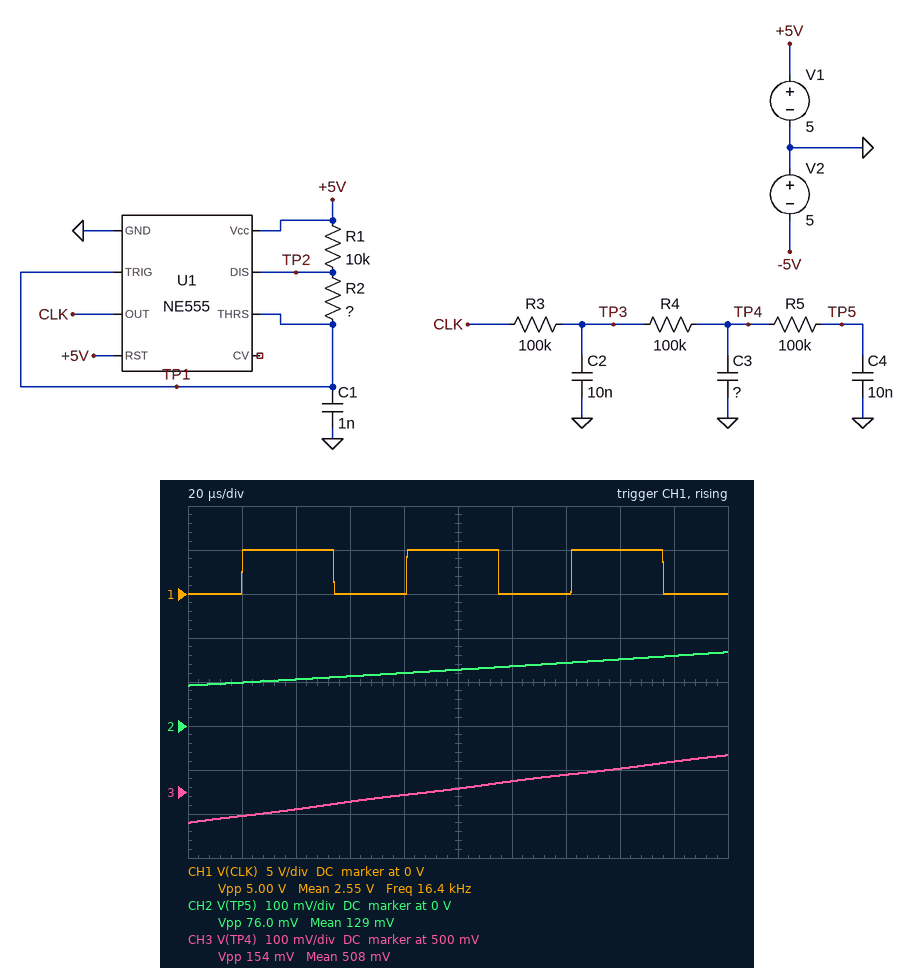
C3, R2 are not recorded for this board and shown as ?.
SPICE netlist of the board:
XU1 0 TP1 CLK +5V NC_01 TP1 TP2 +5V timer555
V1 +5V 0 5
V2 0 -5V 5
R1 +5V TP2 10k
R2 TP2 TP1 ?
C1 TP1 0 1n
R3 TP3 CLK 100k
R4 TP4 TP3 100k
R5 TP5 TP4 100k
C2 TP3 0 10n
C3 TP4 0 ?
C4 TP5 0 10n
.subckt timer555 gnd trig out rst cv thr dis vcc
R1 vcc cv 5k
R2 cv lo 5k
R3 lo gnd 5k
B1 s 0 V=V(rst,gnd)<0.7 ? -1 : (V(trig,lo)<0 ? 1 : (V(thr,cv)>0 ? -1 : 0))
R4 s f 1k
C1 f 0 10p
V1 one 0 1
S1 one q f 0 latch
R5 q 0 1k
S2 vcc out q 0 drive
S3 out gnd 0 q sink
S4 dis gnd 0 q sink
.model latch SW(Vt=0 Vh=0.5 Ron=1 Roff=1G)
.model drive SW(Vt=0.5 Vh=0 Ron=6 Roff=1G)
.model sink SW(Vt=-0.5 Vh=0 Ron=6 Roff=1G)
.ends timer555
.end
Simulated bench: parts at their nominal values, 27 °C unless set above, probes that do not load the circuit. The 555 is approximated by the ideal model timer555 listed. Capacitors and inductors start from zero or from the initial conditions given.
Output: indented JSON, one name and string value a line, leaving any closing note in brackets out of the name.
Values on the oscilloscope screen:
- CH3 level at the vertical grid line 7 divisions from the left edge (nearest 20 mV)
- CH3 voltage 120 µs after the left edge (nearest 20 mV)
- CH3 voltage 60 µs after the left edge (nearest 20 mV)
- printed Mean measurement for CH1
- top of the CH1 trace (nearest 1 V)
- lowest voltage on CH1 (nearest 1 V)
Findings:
{
  "CH3 level at the vertical grid line 7 divisions from the left edge": "540 mV",
  "CH3 voltage 120 µs after the left edge": "520 mV",
  "CH3 voltage 60 µs after the left edge": "480 mV",
  "printed Mean measurement for CH1": "2.55 V",
  "top of the CH1 trace": "5 V",
  "lowest voltage on CH1": "0 V"
}
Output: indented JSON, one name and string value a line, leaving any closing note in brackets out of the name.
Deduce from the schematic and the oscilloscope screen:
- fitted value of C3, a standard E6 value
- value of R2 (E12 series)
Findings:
{
  "fitted value of C3, a standard E6 value": "3.3 nF",
  "value of R2": "39 kΩ"
}
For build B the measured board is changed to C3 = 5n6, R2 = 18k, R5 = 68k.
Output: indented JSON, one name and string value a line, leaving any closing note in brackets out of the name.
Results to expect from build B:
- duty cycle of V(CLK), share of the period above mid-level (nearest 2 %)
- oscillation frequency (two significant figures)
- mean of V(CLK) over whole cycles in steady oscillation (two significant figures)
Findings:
{
  "duty cycle of V(CLK), share of the period above mid-level": "60 %",
  "oscillation frequency": "31 kHz",
  "mean of V(CLK) over whole cycles in steady oscillation": "3.0 V"
}
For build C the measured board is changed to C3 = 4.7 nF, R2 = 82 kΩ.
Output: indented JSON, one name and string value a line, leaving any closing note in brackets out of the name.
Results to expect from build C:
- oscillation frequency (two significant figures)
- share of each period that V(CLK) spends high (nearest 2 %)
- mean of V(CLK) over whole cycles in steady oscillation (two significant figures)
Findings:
{
  "oscillation frequency": "8.3 kHz",
  "share of each period that V(CLK) spends high": "52 %",
  "mean of V(CLK) over whole cycles in steady oscillation": "2.6 V"
}
